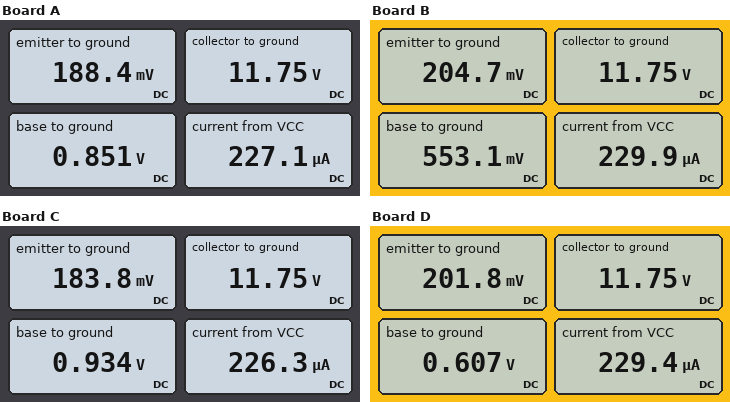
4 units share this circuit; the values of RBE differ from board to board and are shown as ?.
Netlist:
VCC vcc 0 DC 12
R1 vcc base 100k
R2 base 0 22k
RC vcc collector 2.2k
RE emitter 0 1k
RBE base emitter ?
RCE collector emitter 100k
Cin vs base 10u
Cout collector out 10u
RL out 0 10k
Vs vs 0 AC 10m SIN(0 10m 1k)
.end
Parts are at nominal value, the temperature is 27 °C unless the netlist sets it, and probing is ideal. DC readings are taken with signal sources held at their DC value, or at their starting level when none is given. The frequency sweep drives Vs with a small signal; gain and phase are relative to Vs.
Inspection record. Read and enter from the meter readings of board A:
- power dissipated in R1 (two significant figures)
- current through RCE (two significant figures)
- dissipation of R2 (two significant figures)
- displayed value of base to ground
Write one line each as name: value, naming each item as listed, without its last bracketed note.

power dissipated in R1: 1.2 mW
current through RCE: 120 µA
dissipation of R2: 33 µW
displayed value of base to ground: 0.851 V
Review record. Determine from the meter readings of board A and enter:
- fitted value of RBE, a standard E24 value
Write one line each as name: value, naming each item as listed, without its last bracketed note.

fitted value of RBE, a standard E24 value: 9.1 kΩ
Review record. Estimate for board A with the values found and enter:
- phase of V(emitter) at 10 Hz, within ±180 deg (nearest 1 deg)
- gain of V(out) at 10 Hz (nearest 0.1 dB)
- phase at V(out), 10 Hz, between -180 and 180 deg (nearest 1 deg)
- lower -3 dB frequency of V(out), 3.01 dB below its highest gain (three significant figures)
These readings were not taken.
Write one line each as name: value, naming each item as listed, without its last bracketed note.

phase of V(emitter) at 10 Hz, within ±180 deg: 14 deg
gain of V(out) at 10 Hz: -55.5 dB
phase at V(out), 10 Hz, between -180 and 180 deg: 21 deg
lower -3 dB frequency of V(out), 3.01 dB below its highest gain: 2.99 Hz
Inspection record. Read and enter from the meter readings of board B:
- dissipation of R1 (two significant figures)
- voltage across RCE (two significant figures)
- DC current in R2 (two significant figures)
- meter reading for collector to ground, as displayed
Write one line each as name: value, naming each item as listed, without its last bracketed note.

dissipation of R1: 1.3 mW
voltage across RCE: 12 V
DC current in R2: 25 µA
meter reading for collector to ground, as displayed: 11.75 V
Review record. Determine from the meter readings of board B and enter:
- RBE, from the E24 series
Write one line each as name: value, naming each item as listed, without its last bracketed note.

RBE, from the E24 series: 3.9 kΩ
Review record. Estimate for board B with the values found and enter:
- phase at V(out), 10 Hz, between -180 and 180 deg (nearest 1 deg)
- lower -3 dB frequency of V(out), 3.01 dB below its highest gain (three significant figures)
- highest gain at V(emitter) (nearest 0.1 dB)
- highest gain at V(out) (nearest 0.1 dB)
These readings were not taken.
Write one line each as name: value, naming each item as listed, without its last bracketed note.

phase at V(out), 10 Hz, between -180 and 180 deg: 30 deg
lower -3 dB frequency of V(out), 3.01 dB below its highest gain: 4.50 Hz
highest gain at V(emitter): -13.9 dB
highest gain at V(out): -48.9 dB
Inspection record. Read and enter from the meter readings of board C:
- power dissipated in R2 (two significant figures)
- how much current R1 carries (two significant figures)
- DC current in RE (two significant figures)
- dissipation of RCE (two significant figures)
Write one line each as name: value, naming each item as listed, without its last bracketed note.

power dissipated in R2: 40 µW
how much current R1 carries: 110 µA
DC current in RE: 180 µA
dissipation of RCE: 1.3 mW
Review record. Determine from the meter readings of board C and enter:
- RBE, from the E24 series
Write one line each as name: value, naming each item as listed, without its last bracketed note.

RBE, from the E24 series: 11 kΩ
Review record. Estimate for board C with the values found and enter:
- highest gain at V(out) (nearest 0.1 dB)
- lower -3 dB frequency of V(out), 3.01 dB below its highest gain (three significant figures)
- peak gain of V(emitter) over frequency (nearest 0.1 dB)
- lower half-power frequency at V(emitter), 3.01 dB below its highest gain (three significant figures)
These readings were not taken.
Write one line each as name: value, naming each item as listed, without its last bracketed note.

highest gain at V(out): -56.7 dB
lower -3 dB frequency of V(out), 3.01 dB below its highest gain: 2.77 Hz
peak gain of V(emitter) over frequency: -21.7 dB
lower half-power frequency at V(emitter), 3.01 dB below its highest gain: 2.21 Hz
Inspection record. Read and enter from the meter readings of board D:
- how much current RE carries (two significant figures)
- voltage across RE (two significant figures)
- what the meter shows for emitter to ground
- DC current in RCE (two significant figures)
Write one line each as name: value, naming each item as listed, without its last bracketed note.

how much current RE carries: 200 µA
voltage across RE: 200 mV
what the meter shows for emitter to ground: 201.8 mV
DC current in RCE: 120 µA
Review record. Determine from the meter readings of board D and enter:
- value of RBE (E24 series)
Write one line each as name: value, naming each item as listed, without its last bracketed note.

value of RBE: 4.7 kΩ
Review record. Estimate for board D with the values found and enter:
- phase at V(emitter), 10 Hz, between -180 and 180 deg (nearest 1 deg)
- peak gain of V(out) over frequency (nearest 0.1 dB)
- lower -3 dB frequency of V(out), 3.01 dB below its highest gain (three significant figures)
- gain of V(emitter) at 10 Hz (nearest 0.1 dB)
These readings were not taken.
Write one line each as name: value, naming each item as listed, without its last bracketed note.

phase at V(emitter), 10 Hz, between -180 and 180 deg: 20 deg
peak gain of V(out) over frequency: -50.2 dB
lower -3 dB frequency of V(out), 3.01 dB below its highest gain: 4.08 Hz
gain of V(emitter) at 10 Hz: -15.7 dB
